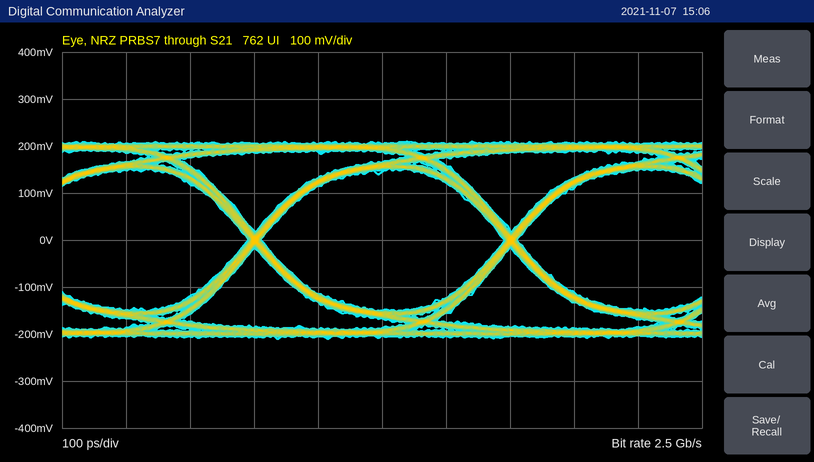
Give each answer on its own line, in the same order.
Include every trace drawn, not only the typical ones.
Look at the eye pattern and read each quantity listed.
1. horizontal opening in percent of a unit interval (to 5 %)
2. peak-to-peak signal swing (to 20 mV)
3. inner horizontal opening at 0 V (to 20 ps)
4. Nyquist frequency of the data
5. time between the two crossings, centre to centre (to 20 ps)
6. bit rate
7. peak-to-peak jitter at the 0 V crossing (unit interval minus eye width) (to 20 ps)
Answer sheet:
95 %
420 mV
380 ps
1.25 GHz
400 ps
2.5 Gb/s
20 ps
